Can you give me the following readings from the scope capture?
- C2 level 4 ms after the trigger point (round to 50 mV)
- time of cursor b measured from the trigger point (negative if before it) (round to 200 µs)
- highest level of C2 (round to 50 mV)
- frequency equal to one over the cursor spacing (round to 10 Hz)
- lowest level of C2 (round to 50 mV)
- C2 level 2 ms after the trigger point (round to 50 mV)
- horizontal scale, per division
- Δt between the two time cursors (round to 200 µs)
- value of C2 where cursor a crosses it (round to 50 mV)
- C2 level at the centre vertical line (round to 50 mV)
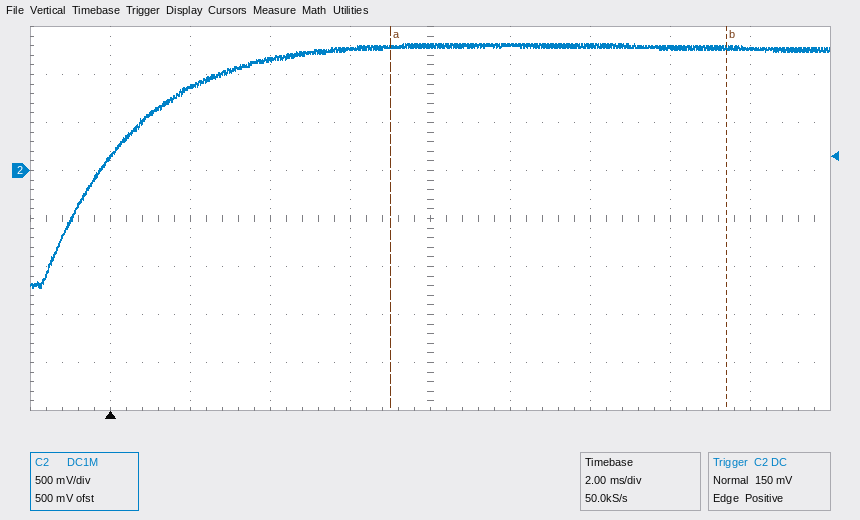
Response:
1.15 V
+15.4 ms
1.30 V
120 Hz
-1.20 V
850 mV
2 ms
8.4 ms
1.30 V
1.30 V
